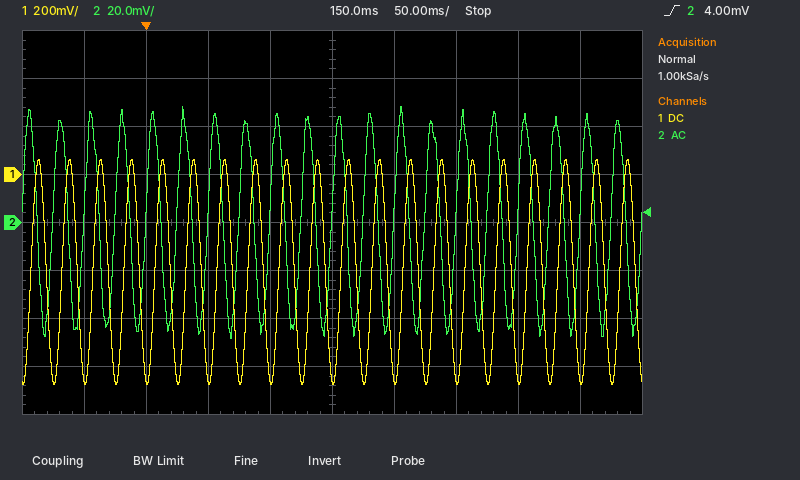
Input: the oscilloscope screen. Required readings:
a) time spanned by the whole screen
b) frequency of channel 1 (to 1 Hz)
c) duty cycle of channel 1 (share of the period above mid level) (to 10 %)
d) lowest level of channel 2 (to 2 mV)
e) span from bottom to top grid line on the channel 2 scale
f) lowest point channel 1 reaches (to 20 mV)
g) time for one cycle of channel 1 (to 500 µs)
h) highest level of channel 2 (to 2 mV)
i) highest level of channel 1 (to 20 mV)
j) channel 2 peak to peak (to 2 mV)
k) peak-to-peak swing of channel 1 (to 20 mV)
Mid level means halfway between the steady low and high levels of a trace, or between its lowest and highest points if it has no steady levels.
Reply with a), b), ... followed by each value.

a) 500 ms
b) 40 Hz
c) 50 %
d) -48 mV
e) 160 mV
f) -880 mV
g) 25.0 ms
h) 48 mV
i) 60 mV
j) 96 mV
k) 940 mV
